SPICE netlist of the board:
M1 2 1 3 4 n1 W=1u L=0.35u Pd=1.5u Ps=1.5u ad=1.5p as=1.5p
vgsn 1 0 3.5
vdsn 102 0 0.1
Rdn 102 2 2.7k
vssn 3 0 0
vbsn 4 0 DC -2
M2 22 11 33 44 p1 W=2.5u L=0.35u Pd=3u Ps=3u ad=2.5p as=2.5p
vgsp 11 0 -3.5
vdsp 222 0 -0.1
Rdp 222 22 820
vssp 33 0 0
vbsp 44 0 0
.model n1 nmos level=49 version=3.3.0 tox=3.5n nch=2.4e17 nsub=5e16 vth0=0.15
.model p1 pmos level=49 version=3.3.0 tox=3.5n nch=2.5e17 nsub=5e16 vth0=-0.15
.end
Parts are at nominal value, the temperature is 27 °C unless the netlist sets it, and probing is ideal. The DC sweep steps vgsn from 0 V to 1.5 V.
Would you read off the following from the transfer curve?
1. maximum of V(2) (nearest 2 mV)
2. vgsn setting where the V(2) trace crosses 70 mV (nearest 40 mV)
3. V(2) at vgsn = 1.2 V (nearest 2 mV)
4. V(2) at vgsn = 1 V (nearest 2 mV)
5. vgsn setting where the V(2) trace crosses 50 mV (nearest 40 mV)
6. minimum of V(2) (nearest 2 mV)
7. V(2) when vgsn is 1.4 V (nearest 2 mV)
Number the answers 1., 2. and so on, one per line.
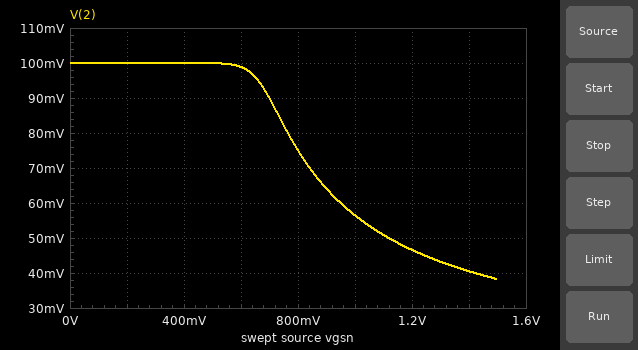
1. 100 mV
2. 840 mV
3. 46 mV
4. 56 mV
5. 1.12 V
6. 38 mV
7. 40 mV
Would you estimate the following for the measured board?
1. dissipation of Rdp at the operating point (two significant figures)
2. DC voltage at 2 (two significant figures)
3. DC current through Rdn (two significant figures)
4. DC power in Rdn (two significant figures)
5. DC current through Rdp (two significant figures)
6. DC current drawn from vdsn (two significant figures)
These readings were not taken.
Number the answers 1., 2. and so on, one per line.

1. 3.2 µW
2. 24 mV
3. 28 µA
4. 2.1 µW
5. 63 µA
6. 28 µA
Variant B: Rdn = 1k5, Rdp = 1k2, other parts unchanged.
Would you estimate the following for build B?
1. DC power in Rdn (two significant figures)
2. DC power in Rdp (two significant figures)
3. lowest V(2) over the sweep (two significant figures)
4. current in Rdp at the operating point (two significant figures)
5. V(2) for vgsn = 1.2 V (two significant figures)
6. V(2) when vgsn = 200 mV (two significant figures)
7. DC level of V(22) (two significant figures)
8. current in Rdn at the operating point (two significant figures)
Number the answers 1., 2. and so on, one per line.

1. 2.7 µW
2. 3.1 µW
3. 53 mV
4. 51 µA
5. 62 mV
6. 100 mV
7. -39 mV
8. 42 µA
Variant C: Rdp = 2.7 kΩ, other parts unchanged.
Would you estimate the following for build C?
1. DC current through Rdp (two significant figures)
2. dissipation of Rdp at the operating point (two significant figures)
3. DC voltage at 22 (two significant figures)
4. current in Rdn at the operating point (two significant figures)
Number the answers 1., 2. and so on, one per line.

1. 29 µA
2. 2.2 µW
3. -22 mV
4. 28 µA
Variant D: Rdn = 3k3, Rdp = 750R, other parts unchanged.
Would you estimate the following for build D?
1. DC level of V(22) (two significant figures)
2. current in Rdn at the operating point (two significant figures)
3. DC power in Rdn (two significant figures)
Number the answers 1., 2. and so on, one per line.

1. -51 mV
2. 24 µA
3. 1.9 µW
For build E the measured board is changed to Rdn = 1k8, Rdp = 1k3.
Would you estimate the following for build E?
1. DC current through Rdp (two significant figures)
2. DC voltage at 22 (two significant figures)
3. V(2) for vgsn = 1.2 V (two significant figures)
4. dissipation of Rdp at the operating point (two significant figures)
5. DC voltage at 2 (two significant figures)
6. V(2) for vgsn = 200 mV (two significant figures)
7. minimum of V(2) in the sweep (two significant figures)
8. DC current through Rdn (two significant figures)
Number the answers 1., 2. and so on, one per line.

1. 48 µA
2. -37 mV
3. 57 mV
4. 3.0 µW
5. 32 mV
6. 100 mV
7. 48 mV
8. 38 µA
